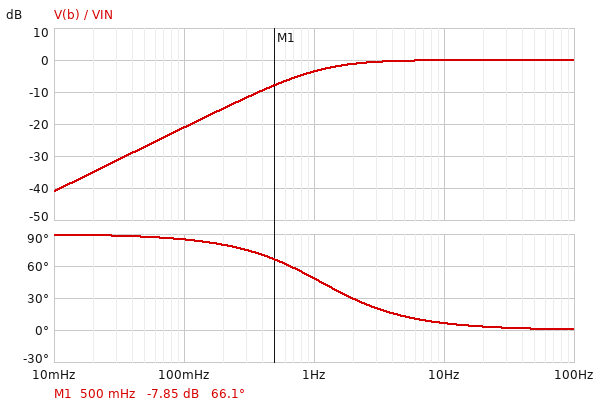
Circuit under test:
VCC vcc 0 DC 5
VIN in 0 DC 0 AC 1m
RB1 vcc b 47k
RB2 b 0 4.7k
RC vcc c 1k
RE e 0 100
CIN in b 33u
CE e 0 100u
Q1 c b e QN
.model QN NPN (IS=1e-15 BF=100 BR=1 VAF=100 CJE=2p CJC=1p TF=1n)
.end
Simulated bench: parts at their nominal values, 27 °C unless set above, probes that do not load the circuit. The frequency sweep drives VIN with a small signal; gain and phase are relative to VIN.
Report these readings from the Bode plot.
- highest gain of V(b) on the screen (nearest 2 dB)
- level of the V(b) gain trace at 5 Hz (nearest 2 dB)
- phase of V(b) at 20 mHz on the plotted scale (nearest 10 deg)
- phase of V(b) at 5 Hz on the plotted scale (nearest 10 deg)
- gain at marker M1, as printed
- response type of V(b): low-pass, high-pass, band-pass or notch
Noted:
0 dB
0 dB
90 deg
10 deg
-7.85 dB
high-pass
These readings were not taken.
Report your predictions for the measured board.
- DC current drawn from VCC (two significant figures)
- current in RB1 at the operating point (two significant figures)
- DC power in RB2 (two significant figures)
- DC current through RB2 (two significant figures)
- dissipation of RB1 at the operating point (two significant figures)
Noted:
97 µA
97 µA
44 µW
97 µA
440 µW
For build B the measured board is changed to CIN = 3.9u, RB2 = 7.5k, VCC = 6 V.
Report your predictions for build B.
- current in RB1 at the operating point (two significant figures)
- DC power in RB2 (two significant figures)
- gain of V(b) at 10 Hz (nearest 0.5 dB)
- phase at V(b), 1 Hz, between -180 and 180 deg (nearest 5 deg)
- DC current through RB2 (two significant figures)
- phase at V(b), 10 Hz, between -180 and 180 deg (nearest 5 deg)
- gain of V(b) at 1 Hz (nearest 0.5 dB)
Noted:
110 µA
81 µW
-3.5 dB
85 deg
100 µA
40 deg
-19.5 dB
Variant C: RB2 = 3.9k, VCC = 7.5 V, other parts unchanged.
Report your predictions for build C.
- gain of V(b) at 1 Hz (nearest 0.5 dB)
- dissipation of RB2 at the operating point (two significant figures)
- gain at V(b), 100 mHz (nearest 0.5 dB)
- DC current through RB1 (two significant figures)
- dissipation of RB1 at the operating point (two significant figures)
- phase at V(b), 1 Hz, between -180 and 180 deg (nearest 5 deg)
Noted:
-4.5 dB
85 µW
-22.5 dB
150 µA
1.0 mW
55 deg
